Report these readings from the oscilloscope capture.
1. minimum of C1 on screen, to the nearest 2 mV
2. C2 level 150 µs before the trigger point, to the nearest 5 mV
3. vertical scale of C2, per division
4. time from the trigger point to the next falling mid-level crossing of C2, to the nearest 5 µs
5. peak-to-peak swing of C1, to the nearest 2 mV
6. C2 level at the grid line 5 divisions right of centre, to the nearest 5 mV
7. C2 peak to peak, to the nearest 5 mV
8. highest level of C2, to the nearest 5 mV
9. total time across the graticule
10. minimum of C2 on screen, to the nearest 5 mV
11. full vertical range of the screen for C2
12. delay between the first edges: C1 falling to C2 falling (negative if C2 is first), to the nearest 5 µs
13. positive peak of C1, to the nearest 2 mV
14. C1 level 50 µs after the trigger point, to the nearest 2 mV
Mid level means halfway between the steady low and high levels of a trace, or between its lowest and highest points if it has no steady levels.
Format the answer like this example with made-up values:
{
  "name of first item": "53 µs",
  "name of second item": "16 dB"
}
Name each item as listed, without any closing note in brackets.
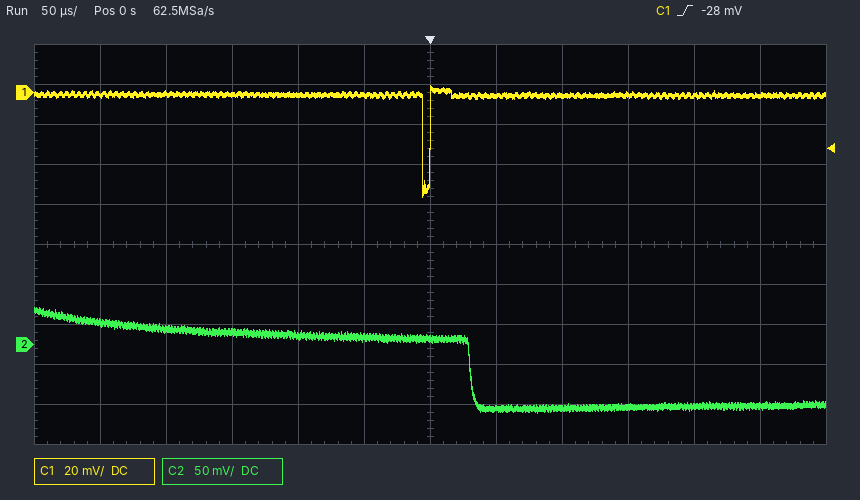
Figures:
{
  "minimum of C1 on screen, to the nearest 2 mV": "-52 mV",
  "C2 level 150 µs before the trigger point, to the nearest 5 mV": "15 mV",
  "vertical scale of C2, per division": "50 mV",
  "time from the trigger point to the next falling mid-level crossing of C2, to the nearest 5 µs": "30 µs",
  "peak-to-peak swing of C1, to the nearest 2 mV": "56 mV",
  "C2 level at the grid line 5 divisions right of centre, to the nearest 5 mV": "-75 mV",
  "C2 peak to peak, to the nearest 5 mV": "130 mV",
  "highest level of C2, to the nearest 5 mV": "45 mV",
  "total time across the graticule": "600 µs",
  "minimum of C2 on screen, to the nearest 5 mV": "-85 mV",
  "full vertical range of the screen for C2": "500 mV",
  "delay between the first edges: C1 falling to C2 falling (negative if C2 is first), to the nearest 5 µs": "+35 µs",
  "positive peak of C1, to the nearest 2 mV": "4 mV",
  "C1 level 50 µs after the trigger point, to the nearest 2 mV": "-2 mV"
}
